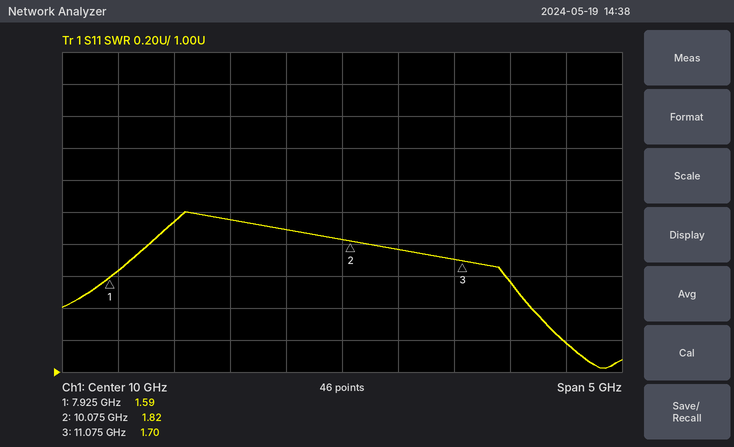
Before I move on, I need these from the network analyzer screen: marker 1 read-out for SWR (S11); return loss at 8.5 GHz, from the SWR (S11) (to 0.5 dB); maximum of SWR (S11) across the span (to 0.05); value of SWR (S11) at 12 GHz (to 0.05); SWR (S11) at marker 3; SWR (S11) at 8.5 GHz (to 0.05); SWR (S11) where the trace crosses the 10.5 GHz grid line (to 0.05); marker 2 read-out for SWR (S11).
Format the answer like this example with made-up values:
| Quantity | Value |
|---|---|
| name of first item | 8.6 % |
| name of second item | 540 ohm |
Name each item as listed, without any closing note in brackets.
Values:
| Quantity | Value |
|---|---|
| marker 1 read-out for SWR | 1.59 |
| return loss at 8.5 GHz, from the SWR (S11) | 10.0 dB |
| maximum of SWR (S11) across the span | 2.00 |
| value of SWR (S11) at 12 GHz | 1.20 |
| SWR (S11) at marker 3 | 1.70 |
| SWR (S11) at 8.5 GHz | 1.95 |
| SWR (S11) where the trace crosses the 10.5 GHz grid line | 1.75 |
| marker 2 read-out for SWR | 1.82 |
